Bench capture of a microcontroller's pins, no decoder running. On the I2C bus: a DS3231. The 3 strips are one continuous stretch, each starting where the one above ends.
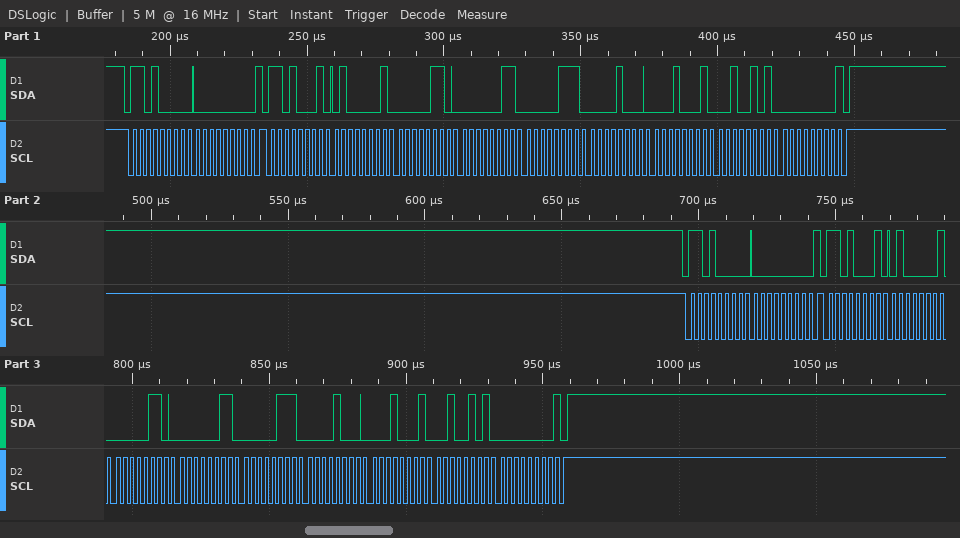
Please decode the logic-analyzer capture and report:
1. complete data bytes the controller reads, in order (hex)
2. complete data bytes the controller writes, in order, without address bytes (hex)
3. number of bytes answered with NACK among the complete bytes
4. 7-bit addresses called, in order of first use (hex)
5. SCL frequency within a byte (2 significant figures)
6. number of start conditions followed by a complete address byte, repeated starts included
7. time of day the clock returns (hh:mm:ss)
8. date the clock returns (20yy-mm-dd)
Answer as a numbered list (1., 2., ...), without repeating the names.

1. 41 06 03 07 08 11 25 00 41 06 03 07 08 11 25 00
2. 00 00
3. 2
4. 0x68
5. 400 kHz
6. 4
7. 03:06:41
8. 2025-11-08
